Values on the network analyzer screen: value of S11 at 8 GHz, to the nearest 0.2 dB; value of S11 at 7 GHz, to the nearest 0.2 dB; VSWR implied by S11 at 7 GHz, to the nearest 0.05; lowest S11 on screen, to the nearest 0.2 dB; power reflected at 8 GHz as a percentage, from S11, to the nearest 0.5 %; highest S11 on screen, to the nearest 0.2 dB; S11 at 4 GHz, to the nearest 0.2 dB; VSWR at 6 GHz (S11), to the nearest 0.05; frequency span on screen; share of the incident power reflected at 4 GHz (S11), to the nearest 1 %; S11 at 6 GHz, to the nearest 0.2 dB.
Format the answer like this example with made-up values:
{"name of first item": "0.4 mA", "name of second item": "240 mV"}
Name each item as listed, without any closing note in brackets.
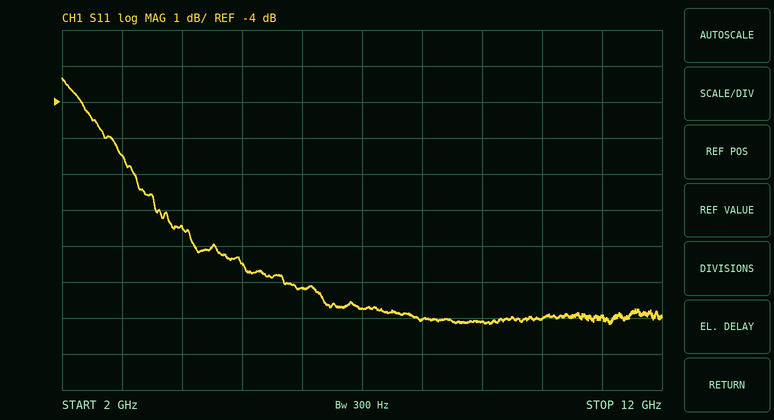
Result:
{"value of S11 at 8 GHz, to the nearest 0.2 dB": "-10.0 dB", "value of S11 at 7 GHz, to the nearest 0.2 dB": "-9.8 dB", "VSWR implied by S11 at 7 GHz, to the nearest 0.05": "1.95", "lowest S11 on screen, to the nearest 0.2 dB": "-10.2 dB", "power reflected at 8 GHz as a percentage, from S11, to the nearest 0.5 %": "10.0 %", "highest S11 on screen, to the nearest 0.2 dB": "-3.4 dB", "S11 at 4 GHz, to the nearest 0.2 dB": "-7.4 dB", "VSWR at 6 GHz (S11), to the nearest 0.05": "2.05", "frequency span on screen": "10 GHz", "share of the incident power reflected at 4 GHz (S11), to the nearest 1 %": "18 %", "S11 at 6 GHz, to the nearest 0.2 dB": "-9.2 dB"}
